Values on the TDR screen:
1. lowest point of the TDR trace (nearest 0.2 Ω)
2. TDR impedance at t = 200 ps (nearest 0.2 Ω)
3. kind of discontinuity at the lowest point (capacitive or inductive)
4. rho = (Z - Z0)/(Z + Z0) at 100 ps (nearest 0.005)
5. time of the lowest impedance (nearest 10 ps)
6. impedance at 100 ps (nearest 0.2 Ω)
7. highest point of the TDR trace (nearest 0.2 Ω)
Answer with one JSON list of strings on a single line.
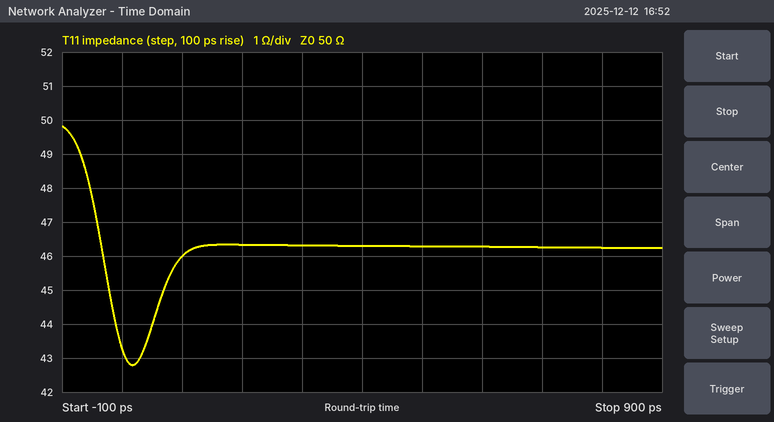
["42.8 Ω", "46.4 Ω", "capacitive", "-0.040", "20 ps", "46.0 Ω", "49.8 Ω"]
